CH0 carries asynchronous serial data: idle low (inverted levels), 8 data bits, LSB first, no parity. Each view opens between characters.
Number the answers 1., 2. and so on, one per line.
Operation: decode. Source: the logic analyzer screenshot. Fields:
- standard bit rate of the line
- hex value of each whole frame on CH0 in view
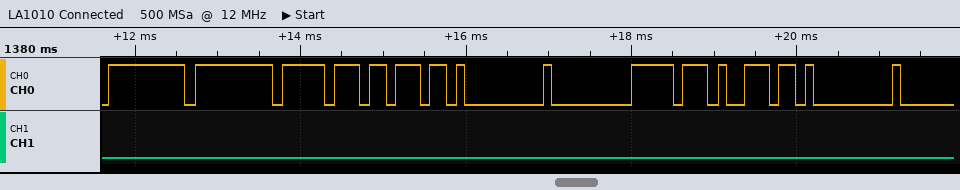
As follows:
1. 9600 baud
2. 00, 00, 10, 22, FF, FF, 10, 23, FF
